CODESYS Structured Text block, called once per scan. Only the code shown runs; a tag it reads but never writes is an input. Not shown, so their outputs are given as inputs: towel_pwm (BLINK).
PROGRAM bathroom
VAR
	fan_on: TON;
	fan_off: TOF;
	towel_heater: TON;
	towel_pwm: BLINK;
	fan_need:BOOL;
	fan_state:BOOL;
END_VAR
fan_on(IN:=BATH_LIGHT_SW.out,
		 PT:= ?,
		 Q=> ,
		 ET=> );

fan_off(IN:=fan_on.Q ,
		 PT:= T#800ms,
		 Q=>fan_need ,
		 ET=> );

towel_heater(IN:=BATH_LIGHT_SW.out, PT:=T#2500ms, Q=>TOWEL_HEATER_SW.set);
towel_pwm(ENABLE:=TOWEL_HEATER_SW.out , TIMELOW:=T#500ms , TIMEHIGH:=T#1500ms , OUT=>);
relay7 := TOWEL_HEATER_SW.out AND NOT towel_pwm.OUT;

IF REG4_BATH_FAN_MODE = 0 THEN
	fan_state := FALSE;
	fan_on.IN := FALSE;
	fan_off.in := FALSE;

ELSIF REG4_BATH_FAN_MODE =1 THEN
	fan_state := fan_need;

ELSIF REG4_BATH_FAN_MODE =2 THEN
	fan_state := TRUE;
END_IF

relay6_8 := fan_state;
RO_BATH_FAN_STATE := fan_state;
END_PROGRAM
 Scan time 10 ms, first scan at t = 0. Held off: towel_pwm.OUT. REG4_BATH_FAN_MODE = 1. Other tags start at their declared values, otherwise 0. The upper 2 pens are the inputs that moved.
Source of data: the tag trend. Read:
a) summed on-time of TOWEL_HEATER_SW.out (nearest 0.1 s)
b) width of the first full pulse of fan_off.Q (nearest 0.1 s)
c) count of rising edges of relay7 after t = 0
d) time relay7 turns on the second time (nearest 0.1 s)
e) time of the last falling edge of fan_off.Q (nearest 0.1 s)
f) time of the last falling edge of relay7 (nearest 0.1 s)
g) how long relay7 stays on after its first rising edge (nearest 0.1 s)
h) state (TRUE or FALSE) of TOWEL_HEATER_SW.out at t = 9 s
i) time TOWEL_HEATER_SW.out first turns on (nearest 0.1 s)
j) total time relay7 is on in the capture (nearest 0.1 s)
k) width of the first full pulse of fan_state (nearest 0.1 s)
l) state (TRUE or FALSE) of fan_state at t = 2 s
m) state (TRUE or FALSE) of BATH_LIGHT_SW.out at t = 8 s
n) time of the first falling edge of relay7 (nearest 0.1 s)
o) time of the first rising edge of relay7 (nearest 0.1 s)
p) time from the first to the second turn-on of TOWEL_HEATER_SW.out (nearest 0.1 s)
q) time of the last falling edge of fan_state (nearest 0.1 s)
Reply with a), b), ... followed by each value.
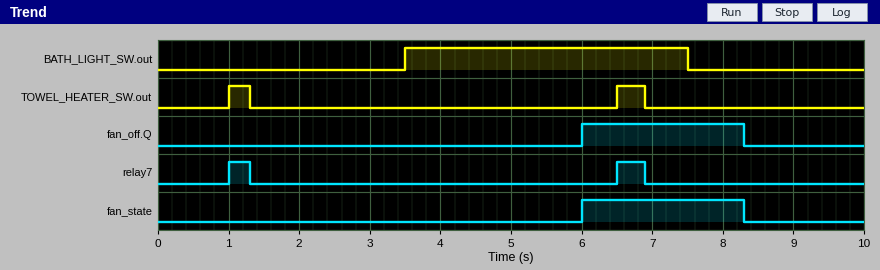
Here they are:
a) 0.7 s
b) 2.3 s
c) 2
d) 6.5 s
e) 8.3 s
f) 6.9 s
g) 0.3 s
h) FALSE
i) 1.0 s
j) 0.7 s
k) 2.3 s
l) FALSE
m) FALSE
n) 1.3 s
o) 1.0 s
p) 5.5 s
q) 8.3 s
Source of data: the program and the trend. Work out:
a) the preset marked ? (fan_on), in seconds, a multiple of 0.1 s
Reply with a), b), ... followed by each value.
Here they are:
a) 2.5 s
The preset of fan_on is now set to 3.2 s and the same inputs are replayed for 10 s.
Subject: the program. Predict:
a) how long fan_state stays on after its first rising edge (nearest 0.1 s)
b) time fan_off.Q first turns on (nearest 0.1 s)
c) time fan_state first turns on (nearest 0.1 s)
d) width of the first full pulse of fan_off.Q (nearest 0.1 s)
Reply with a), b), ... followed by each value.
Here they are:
a) 1.6 s
b) 6.7 s
c) 6.7 s
d) 1.6 s
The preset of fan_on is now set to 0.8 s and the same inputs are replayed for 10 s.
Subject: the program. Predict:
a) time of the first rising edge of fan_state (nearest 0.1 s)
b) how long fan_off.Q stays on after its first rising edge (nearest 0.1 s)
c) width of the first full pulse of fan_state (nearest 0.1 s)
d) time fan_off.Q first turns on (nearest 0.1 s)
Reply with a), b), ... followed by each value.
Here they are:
a) 4.3 s
b) 4.0 s
c) 4.0 s
d) 4.3 s
